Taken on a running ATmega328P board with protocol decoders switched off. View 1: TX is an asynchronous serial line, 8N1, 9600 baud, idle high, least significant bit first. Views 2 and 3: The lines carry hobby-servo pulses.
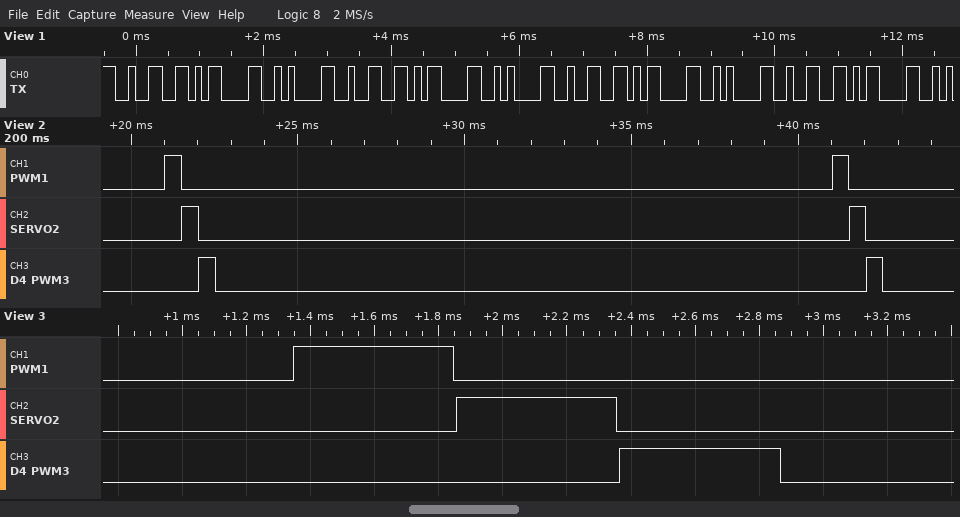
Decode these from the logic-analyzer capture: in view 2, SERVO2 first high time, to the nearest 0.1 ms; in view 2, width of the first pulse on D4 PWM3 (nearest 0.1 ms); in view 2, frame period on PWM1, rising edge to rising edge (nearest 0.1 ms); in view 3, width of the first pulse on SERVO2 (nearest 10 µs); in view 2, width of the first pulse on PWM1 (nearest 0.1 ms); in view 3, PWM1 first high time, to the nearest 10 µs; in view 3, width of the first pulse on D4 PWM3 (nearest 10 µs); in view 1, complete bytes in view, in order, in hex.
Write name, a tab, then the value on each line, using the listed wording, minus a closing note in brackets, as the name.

in view 2, SERVO2 first high time, to the nearest 0.1 ms	0.5 ms
in view 2, width of the first pulse on D4 PWM3	0.5 ms
in view 2, frame period on PWM1, rising edge to rising edge	20.0 ms
in view 3, width of the first pulse on SERVO2	500 µs
in view 2, width of the first pulse on PWM1	0.5 ms
in view 3, PWM1 first high time, to the nearest 10 µs	500 µs
in view 3, width of the first pulse on D4 PWM3	500 µs
in view 1, complete bytes in view, in order, in hex	0x32 0x0D 0x0A 0x32 0x0D 0x0A 0x32 0x0D 0x0A 0x32 0x0D
